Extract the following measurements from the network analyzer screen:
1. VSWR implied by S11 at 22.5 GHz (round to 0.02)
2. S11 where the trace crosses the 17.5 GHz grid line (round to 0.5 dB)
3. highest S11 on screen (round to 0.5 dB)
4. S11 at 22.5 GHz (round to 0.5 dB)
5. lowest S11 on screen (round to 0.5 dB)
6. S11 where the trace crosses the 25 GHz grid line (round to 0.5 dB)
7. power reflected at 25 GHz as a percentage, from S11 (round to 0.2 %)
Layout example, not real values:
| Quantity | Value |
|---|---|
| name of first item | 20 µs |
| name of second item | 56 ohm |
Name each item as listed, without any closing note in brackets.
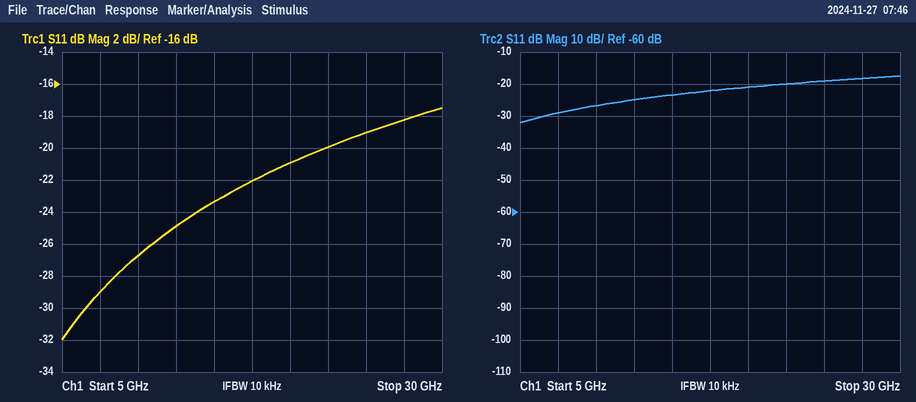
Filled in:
| Quantity | Value |
|---|---|
| VSWR implied by S11 at 22.5 GHz | 1.22 |
| S11 where the trace crosses the 17.5 GHz grid line | -22.0 dB |
| highest S11 on screen | -17.5 dB |
| S11 at 22.5 GHz | -20.0 dB |
| lowest S11 on screen | -32.0 dB |
| S11 where the trace crosses the 25 GHz grid line | -19.0 dB |
| power reflected at 25 GHz as a percentage, from S11 | 1.2 % |
